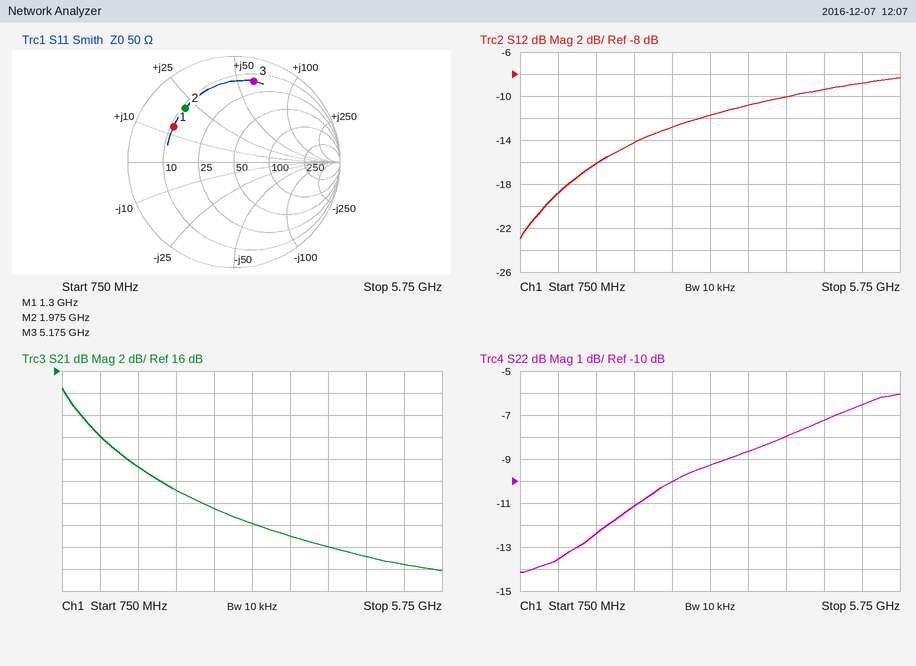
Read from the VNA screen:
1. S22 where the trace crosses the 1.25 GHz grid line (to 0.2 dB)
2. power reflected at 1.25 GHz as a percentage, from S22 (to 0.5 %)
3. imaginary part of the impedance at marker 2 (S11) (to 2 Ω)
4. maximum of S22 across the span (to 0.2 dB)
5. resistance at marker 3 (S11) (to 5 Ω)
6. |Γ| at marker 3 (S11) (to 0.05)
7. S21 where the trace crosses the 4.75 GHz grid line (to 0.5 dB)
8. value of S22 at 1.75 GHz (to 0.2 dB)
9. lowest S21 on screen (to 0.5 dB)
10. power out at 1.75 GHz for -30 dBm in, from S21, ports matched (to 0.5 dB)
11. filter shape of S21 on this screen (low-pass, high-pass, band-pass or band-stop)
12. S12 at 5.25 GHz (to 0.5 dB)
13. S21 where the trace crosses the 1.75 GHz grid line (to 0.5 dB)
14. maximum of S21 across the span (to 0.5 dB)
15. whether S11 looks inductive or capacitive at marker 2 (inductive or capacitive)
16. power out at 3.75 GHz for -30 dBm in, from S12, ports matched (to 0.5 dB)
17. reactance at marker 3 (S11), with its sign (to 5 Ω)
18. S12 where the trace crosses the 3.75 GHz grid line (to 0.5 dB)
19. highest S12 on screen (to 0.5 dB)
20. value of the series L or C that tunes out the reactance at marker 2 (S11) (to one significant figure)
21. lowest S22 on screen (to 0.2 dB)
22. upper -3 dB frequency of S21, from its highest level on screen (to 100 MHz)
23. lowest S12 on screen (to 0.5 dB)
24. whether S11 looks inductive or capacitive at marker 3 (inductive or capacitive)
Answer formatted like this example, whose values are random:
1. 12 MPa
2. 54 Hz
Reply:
1. -13.6 dB
2. 4.5 %
3. +22 Ω
4. -6.0 dB
5. 15 Ω
6. 0.80
7. -1.0 dB
8. -12.4 dB
9. -2.0 dB
10. -22.5 dBm
11. low-pass
12. -9.0 dB
13. 7.5 dB
14. 14.5 dB
15. inductive
16. -41.0 dBm
17. +60 Ω
18. -11.0 dB
19. -8.5 dB
20. 4 pF
21. -14.2 dB
22. 1.1 GHz
23. -23.0 dB
24. inductive
